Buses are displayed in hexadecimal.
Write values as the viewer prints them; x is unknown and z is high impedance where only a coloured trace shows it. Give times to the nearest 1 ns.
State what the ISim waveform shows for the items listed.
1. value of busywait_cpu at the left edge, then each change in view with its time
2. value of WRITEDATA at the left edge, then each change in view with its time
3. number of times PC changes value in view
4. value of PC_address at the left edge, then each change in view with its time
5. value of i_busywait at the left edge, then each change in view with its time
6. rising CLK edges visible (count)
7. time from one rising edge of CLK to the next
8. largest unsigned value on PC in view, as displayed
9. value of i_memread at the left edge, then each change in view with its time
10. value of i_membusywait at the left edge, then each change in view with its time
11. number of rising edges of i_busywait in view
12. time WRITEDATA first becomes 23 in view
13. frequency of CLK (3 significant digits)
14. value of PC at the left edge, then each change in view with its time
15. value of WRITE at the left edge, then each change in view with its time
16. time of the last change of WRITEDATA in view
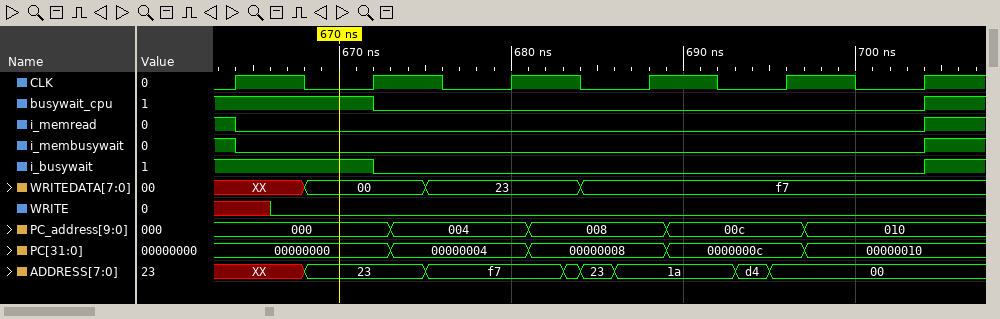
1, 0 at 672 ns, 1 at 704 ns
XX, 00 at 668 ns, 23 at 675 ns, f7 at 684 ns
4
000, 004 at 673 ns, 008 at 681 ns, 00c at 689 ns, 010 at 697 ns
1, 0 at 672 ns, 1 at 704 ns
6
8 ns
00000010
1, 0 at 664 ns, 1 at 704 ns
1, 0 at 664 ns, 1 at 704 ns
1
675 ns
125 MHz
00000000, 00000004 at 673 ns, 00000008 at 681 ns, 0000000c at 689 ns, 00000010 at 697 ns
x, 0 at 666 ns
684 ns
